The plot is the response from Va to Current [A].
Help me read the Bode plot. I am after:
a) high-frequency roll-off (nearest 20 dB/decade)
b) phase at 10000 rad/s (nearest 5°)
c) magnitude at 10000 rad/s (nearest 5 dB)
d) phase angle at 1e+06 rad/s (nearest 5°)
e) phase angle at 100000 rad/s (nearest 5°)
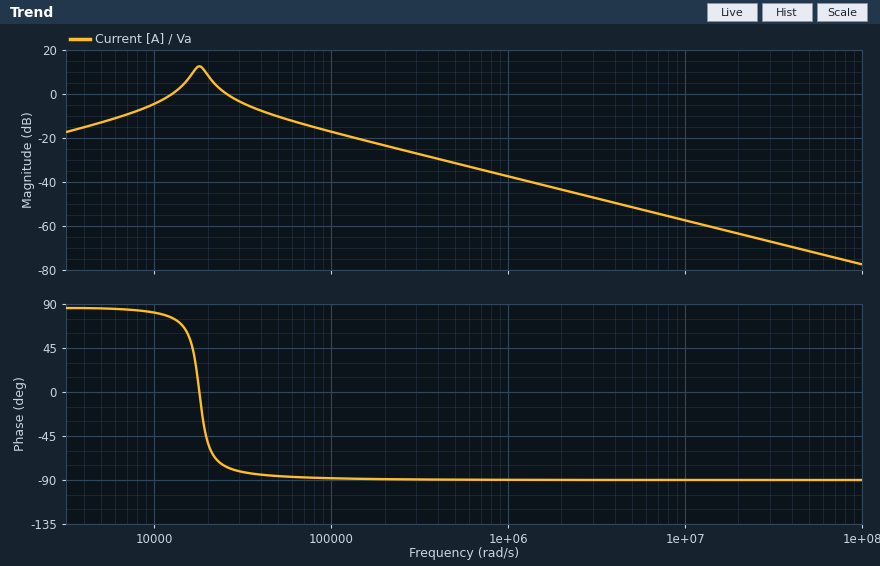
-20 dB/decade
80°
-5 dB
-90°
-90°
